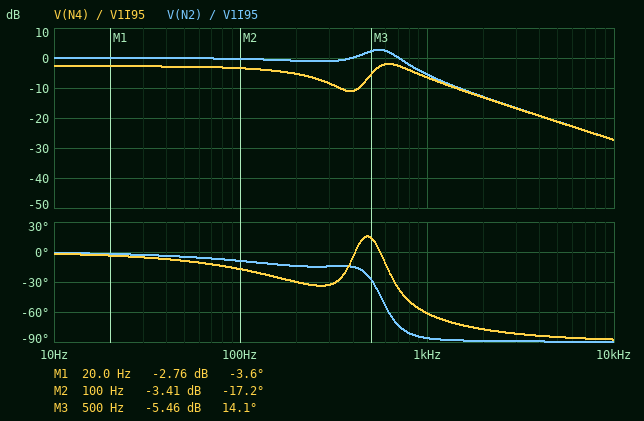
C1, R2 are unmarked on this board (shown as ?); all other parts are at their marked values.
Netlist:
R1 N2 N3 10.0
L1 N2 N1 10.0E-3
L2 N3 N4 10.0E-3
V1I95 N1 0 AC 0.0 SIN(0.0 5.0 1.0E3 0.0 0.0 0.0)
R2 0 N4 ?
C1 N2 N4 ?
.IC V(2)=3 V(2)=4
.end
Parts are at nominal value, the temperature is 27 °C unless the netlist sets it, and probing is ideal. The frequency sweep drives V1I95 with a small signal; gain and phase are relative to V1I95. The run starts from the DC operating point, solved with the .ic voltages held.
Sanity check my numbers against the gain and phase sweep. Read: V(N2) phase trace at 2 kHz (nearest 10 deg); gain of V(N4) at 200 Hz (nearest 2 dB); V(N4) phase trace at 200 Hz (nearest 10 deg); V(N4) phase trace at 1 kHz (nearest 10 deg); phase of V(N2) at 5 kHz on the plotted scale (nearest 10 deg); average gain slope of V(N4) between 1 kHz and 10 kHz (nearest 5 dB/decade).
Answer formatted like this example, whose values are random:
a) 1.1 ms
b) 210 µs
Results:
a) -90 deg
b) -6 dB
c) -30 deg
d) -60 deg
e) -90 deg
f) -20 dB/decade
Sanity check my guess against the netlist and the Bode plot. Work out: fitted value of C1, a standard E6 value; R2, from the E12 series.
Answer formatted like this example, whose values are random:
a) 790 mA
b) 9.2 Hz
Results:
a) 15 µF
b) 27 Ω
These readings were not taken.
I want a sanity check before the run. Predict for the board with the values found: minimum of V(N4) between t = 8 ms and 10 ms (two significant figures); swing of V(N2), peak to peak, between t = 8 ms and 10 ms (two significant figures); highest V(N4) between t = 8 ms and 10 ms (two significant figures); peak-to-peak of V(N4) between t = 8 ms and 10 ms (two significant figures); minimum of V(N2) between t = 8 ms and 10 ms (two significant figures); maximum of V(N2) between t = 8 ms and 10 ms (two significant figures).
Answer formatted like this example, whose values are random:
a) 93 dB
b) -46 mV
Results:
a) -2.4 V
b) 5.3 V
c) 2.4 V
d) 4.7 V
e) -2.6 V
f) 2.6 V
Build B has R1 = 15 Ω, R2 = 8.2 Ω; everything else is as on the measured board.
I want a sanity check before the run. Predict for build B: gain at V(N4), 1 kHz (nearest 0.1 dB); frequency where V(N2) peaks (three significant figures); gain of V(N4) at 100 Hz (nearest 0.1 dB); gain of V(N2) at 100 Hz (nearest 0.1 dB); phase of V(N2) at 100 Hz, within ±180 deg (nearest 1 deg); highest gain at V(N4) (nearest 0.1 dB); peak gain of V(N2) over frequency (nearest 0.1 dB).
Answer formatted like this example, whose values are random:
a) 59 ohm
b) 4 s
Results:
a) -15.9 dB
b) 563 Hz
c) -10.3 dB
d) -0.6 dB
e) -13 deg
f) -7.1 dB
g) 5.3 dB
